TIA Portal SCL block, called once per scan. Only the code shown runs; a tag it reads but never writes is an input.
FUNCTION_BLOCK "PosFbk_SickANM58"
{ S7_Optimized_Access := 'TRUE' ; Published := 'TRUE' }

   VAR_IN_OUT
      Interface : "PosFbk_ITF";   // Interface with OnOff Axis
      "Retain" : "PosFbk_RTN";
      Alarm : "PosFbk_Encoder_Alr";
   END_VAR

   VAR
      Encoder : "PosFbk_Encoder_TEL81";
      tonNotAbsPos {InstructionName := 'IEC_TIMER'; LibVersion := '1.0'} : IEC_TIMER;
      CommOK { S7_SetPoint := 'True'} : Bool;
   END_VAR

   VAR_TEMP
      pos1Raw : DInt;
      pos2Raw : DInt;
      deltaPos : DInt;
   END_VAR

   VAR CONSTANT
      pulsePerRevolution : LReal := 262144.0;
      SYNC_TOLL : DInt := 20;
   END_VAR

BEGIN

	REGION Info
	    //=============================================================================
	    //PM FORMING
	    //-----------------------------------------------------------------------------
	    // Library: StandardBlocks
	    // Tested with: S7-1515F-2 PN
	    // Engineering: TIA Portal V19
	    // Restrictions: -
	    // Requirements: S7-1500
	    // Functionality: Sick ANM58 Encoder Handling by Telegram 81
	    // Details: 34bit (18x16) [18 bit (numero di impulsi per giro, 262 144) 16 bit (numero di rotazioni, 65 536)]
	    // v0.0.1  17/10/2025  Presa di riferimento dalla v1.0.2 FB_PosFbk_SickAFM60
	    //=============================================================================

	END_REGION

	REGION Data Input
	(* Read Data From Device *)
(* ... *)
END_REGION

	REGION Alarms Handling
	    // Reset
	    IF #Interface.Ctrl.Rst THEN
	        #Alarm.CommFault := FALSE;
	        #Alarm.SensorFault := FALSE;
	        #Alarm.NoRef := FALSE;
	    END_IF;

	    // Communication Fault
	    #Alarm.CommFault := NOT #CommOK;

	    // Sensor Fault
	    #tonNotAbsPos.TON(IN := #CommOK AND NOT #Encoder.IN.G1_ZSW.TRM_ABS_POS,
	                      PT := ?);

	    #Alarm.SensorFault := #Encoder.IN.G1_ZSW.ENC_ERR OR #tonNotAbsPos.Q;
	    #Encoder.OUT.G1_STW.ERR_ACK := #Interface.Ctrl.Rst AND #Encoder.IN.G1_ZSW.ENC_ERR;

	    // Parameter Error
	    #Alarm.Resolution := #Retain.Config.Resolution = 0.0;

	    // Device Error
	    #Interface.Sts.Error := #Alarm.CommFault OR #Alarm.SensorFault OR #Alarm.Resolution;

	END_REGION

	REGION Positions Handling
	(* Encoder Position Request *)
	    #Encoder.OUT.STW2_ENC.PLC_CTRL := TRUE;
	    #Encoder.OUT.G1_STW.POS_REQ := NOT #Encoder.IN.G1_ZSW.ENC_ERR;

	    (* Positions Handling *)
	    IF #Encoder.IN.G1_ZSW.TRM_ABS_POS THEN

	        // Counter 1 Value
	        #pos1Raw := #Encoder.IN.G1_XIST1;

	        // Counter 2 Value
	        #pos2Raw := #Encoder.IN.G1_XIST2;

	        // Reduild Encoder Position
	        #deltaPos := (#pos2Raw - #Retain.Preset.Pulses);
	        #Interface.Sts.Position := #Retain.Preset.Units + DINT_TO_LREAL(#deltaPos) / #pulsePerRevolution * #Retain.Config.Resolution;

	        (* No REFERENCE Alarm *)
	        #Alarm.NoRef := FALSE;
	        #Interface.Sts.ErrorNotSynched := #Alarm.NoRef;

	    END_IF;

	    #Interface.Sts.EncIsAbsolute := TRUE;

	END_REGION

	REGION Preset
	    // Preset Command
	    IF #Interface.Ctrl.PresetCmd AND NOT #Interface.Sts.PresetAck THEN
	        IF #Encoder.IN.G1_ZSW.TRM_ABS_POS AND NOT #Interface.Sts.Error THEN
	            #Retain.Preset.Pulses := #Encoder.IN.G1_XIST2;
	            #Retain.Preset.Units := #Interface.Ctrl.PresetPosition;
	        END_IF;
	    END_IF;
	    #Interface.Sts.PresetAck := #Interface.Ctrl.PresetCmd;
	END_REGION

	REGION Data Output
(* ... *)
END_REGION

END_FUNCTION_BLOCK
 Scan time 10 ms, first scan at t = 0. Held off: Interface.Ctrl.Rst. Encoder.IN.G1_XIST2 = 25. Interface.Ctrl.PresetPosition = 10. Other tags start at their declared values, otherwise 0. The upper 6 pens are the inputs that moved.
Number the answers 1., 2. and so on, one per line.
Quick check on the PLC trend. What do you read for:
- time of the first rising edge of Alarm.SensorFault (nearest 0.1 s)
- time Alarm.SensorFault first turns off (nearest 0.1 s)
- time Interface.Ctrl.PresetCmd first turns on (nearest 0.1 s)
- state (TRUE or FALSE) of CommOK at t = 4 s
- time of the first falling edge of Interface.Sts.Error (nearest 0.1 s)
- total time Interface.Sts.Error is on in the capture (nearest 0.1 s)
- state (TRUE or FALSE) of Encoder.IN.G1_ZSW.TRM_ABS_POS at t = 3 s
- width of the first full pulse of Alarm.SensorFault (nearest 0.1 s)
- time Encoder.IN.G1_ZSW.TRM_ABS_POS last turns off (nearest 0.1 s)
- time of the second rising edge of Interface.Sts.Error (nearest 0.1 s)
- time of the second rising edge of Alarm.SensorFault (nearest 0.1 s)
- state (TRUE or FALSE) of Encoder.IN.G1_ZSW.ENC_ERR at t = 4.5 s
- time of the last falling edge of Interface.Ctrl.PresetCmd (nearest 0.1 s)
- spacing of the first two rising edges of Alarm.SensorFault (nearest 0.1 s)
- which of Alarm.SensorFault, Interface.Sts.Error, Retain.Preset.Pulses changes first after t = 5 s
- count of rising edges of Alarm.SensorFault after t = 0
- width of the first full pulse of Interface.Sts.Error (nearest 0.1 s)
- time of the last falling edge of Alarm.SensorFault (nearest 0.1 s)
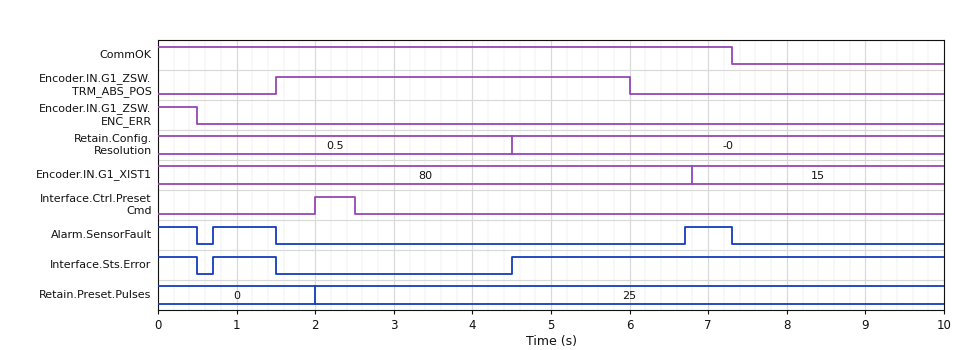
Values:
1. 0.7 s
2. 0.5 s
3. 2.0 s
4. TRUE
5. 0.5 s
6. 6.8 s
7. TRUE
8. 0.8 s
9. 6.0 s
10. 4.5 s
11. 6.7 s
12. FALSE
13. 2.5 s
14. 6.0 s
15. Alarm.SensorFault
16. 2
17. 0.8 s
18. 7.3 s
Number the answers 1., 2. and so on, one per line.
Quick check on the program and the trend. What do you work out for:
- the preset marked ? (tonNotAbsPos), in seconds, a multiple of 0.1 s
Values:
1. 0.7 s
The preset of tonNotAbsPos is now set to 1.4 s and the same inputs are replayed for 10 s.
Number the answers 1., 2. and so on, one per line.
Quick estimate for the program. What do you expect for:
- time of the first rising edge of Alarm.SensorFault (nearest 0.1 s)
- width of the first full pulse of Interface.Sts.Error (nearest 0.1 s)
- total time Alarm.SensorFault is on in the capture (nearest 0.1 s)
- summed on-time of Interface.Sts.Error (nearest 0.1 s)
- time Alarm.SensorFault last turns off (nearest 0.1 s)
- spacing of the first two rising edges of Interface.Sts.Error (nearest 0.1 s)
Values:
1. 1.4 s
2. 0.1 s
3. 0.6 s
4. 6.1 s
5. 1.5 s
6. 3.1 s
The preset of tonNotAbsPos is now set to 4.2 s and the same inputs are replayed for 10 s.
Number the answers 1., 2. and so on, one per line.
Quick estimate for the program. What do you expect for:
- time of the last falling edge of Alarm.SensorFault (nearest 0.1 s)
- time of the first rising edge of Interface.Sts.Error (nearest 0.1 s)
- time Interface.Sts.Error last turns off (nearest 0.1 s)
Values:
1. 0.5 s
2. 4.5 s
3. 0.5 s
